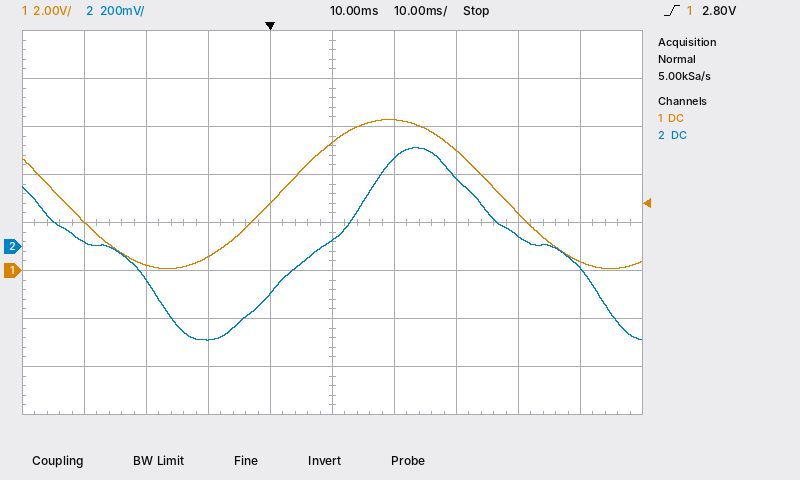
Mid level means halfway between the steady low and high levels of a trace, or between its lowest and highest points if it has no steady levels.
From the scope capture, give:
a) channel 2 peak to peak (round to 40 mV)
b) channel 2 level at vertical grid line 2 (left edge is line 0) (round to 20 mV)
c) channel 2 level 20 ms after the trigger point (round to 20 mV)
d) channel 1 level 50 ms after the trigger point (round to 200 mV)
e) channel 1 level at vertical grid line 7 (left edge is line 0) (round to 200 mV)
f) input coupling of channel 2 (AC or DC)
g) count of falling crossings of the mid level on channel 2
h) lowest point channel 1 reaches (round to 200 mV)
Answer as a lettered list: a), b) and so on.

a) 800 mV
b) -140 mV
c) 360 mV
d) 400 mV
e) 5.0 V
f) DC
g) 2
h) 0.0 V
